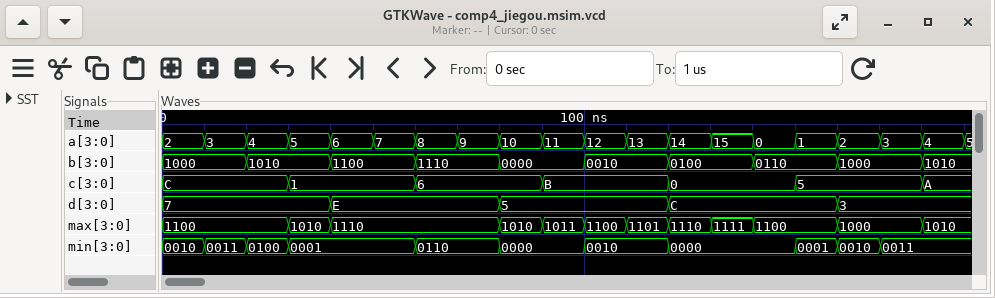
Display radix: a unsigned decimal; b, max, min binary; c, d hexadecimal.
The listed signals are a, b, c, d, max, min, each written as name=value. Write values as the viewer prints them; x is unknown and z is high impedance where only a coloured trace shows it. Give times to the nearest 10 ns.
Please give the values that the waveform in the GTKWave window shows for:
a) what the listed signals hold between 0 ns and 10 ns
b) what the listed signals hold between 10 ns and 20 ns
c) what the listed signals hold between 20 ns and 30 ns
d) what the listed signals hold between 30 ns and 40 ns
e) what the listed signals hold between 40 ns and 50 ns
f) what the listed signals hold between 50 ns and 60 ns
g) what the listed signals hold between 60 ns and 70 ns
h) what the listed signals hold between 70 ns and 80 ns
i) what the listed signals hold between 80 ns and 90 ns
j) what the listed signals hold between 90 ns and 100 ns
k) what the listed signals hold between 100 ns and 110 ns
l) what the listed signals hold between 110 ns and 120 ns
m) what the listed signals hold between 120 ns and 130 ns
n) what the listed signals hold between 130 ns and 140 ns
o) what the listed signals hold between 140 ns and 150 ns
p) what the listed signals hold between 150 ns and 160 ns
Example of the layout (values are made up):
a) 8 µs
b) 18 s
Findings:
a) a=2, b=1000, c=C, d=7, max=1100, min=0010
b) a=3, b=1000, c=C, d=7, max=1100, min=0011
c) a=4, b=1010, c=C, d=7, max=1100, min=0100
d) a=5, b=1010, c=1, d=7, max=1010, min=0001
e) a=6, b=1100, c=1, d=E, max=1110, min=0001
f) a=7, b=1100, c=1, d=E, max=1110, min=0001
g) a=8, b=1110, c=6, d=E, max=1110, min=0110
h) a=9, b=1110, c=6, d=E, max=1110, min=0110
i) a=10, b=0000, c=6, d=5, max=1010, min=0000
j) a=11, b=0000, c=B, d=5, max=1011, min=0000
k) a=12, b=0010, c=B, d=5, max=1100, min=0010
l) a=13, b=0010, c=B, d=5, max=1101, min=0010
m) a=14, b=0100, c=0, d=C, max=1110, min=0000
n) a=15, b=0100, c=0, d=C, max=1111, min=0000
o) a=0, b=0110, c=0, d=C, max=1100, min=0000
p) a=1, b=0110, c=5, d=C, max=1100, min=0001
